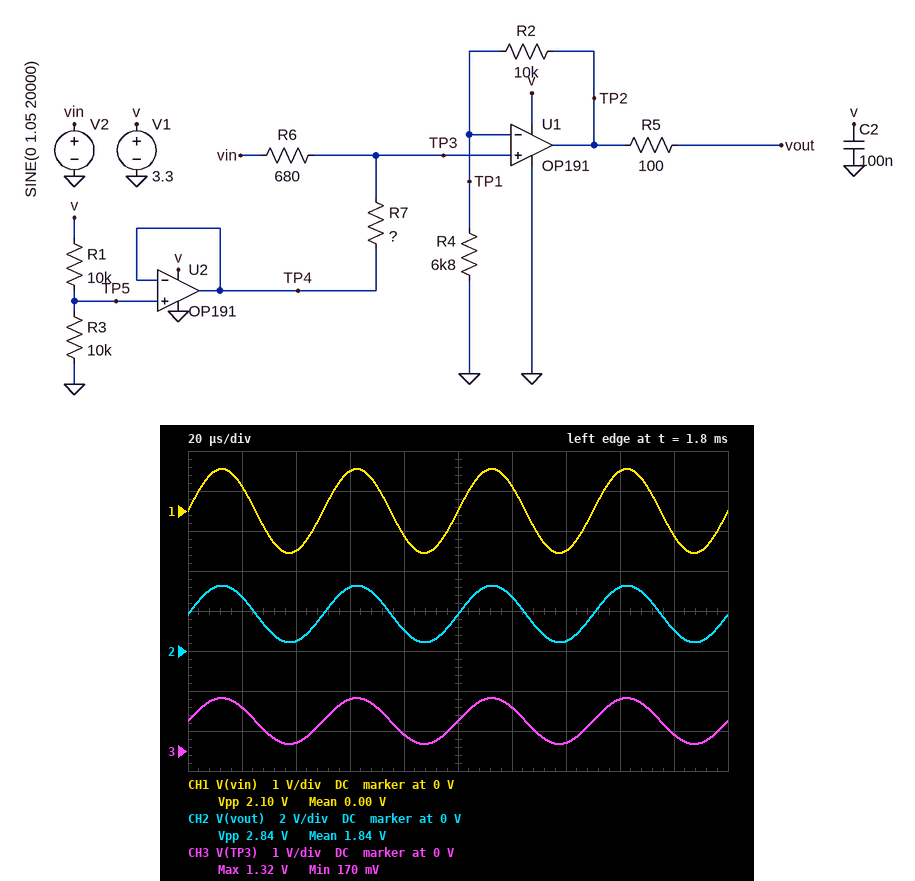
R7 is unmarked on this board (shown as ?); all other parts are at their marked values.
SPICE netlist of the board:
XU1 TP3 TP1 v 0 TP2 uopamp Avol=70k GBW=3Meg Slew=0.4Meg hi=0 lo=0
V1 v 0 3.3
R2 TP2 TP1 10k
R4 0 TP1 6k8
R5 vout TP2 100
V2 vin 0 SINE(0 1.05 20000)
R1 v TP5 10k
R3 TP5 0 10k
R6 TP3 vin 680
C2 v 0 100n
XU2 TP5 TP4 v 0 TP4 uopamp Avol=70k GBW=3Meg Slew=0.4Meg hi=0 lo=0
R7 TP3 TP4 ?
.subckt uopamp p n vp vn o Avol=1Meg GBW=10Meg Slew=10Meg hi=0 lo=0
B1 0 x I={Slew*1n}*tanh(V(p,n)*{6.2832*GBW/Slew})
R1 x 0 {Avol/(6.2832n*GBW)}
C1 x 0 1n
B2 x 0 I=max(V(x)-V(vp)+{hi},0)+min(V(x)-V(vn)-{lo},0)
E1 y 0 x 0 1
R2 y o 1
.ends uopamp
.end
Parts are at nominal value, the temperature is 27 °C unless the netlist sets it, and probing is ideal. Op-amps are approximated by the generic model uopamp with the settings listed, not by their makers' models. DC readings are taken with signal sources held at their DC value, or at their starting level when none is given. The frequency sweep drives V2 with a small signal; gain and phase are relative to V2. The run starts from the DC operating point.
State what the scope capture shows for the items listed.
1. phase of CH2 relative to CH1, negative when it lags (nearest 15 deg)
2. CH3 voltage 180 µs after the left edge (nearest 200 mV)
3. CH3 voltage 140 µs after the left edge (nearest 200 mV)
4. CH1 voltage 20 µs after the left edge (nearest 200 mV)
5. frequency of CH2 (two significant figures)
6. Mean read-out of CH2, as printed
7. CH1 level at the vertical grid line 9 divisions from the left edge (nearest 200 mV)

0 deg
400 mV
200 mV
600 mV
20 kHz
1.84 V
-600 mV
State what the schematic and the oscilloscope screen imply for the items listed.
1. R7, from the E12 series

820 Ω
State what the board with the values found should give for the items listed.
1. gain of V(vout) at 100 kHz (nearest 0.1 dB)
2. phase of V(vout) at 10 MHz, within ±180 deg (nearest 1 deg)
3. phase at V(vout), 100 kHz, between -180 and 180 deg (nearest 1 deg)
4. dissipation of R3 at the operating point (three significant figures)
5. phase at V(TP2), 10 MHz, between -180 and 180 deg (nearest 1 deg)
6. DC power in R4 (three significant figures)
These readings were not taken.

2.6 dB
-83 deg
-5 deg
272 µW
-83 deg
82.3 µW
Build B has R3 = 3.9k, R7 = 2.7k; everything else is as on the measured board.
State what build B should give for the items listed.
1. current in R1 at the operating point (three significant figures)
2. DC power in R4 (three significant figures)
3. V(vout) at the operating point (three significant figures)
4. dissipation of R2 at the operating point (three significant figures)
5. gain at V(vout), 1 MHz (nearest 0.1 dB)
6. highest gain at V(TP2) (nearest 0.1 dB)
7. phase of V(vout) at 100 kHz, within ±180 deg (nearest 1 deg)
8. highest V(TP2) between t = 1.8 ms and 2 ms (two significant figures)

237 µA
5.10 µW
460 mV
7.50 µW
3.7 dB
5.9 dB
-5 deg
2.5 V
